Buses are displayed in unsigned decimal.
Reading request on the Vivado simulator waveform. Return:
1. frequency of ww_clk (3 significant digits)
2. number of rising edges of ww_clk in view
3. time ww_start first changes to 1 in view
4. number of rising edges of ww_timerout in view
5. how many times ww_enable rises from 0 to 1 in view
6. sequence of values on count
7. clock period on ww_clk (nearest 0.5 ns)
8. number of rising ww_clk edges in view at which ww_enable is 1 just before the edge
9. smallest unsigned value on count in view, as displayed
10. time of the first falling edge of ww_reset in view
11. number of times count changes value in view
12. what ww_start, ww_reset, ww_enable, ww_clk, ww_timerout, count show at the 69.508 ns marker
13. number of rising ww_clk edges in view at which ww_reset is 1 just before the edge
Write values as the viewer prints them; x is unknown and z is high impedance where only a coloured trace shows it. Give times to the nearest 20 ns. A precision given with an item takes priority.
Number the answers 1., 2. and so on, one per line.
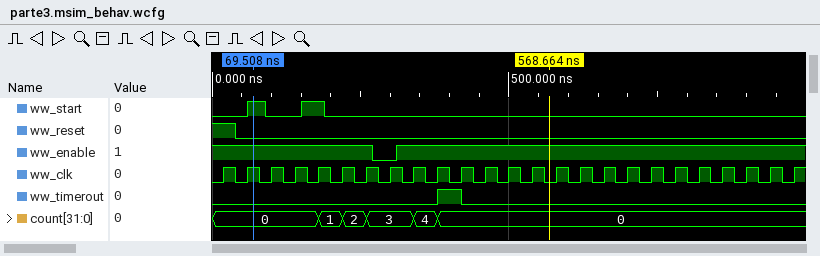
1. 25.0 MHz
2. 25
3. 60 ns
4. 1
5. 1
6. 0, 1, 2, 3, 4, 0
7. 40 ns
8. 24
9. 0
10. 40 ns
11. 5
12. ww_start=1, ww_reset=0, ww_enable=1, ww_clk=1, ww_timerout=0, count=0
13. 1
